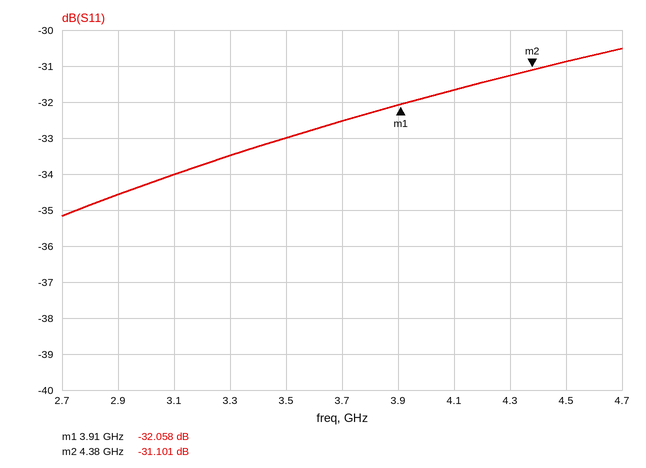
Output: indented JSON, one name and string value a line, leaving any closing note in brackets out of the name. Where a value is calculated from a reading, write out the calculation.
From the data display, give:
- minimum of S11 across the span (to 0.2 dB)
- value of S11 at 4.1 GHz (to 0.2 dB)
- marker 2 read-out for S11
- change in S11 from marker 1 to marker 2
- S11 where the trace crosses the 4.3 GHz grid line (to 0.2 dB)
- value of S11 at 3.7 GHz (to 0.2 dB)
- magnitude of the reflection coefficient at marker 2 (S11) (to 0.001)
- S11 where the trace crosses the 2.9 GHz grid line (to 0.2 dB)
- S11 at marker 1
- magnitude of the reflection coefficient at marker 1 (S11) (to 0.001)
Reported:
{
  "minimum of S11 across the span": "-35.2 dB",
  "value of S11 at 4.1 GHz": "-31.6 dB",
  "marker 2 read-out for S11": "-31.101 dB",
  "change in S11 from marker 1 to marker 2": "-31.101 − (-32.058) = 0.957 dB",
  "S11 where the trace crosses the 4.3 GHz grid line": "-31.2 dB",
  "value of S11 at 3.7 GHz": "-32.6 dB",
  "magnitude of the reflection coefficient at marker 2 (S11)": "10^(-31.101/20) ≈ 0.028",
  "S11 where the trace crosses the 2.9 GHz grid line": "-34.6 dB",
  "S11 at marker 1": "-32.058 dB",
  "magnitude of the reflection coefficient at marker 1 (S11)": "10^(-32.058/20) ≈ 0.025"
}
